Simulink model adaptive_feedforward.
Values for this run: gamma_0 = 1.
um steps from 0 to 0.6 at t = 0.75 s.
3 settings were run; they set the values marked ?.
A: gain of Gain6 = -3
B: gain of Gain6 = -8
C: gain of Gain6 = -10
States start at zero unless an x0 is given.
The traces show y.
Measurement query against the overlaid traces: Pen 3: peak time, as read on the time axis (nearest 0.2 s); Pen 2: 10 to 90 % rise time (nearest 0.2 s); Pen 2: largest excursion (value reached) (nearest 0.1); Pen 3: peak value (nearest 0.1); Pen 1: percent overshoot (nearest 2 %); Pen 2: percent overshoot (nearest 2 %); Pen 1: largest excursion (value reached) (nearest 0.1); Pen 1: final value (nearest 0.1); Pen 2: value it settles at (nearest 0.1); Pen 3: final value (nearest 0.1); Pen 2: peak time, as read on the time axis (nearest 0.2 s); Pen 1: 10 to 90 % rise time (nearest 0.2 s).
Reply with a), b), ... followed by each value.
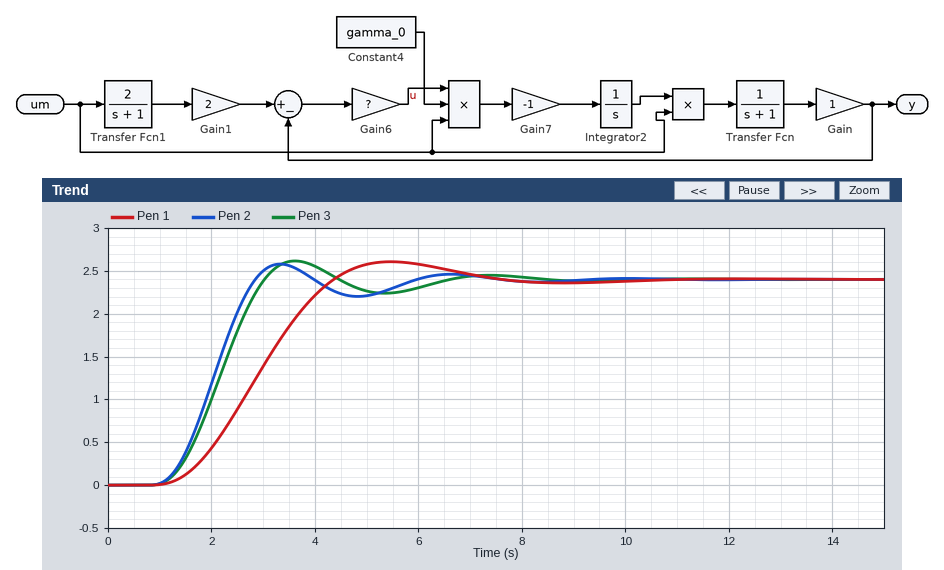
a) 3.6 s
b) 1.2 s
c) 2.6
d) 2.6
e) 8 %
f) 8 %
g) 2.6
h) 2.4
i) 2.4
j) 2.4
k) 3.4 s
l) 2.2 s
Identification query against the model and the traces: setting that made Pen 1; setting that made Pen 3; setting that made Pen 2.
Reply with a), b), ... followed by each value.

a) A
b) B
c) C
